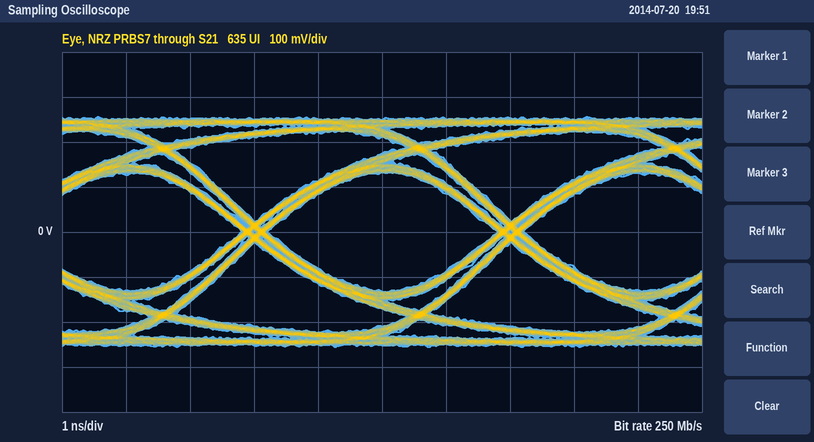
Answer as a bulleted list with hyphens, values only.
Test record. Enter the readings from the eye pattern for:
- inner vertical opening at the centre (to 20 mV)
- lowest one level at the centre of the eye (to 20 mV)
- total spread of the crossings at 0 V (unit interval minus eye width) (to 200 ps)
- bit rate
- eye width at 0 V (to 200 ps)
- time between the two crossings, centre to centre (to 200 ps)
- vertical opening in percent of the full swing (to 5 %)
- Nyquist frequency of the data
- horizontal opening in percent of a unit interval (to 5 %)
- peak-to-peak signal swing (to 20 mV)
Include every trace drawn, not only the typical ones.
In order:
- 260 mV
- 140 mV
- 400 ps
- 250 Mb/s
- 3.6 ns
- 4.0 ns
- 50 %
- 125 MHz
- 90 %
- 520 mV
